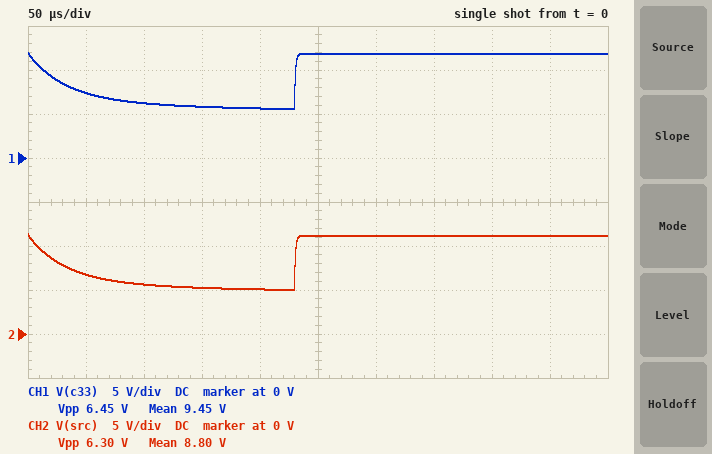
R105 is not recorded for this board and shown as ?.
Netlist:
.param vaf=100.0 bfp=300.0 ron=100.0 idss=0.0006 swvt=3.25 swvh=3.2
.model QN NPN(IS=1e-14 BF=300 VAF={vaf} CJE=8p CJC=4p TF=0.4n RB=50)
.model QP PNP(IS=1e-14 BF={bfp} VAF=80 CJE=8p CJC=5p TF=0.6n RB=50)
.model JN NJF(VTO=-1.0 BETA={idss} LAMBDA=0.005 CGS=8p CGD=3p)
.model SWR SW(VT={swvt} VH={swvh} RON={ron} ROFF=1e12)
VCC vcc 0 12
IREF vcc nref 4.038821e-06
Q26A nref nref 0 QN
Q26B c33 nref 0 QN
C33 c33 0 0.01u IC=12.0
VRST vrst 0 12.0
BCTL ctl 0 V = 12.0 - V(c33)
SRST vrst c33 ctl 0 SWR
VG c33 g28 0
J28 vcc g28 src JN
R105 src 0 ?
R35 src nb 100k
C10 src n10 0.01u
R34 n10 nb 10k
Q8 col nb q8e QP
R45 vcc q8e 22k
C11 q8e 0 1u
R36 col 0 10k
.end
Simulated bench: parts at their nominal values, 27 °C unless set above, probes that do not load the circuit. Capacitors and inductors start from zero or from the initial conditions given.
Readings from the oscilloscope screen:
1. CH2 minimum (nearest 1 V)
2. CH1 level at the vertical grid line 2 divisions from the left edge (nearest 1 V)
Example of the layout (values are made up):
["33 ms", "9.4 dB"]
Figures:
["5 V", "6 V"]
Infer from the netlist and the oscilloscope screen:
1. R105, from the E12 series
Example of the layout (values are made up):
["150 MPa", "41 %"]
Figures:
["3.3 kΩ"]
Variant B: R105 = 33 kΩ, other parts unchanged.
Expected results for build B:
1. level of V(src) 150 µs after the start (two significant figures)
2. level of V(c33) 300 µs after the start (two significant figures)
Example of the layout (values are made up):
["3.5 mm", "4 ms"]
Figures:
["12 V", "12 V"]
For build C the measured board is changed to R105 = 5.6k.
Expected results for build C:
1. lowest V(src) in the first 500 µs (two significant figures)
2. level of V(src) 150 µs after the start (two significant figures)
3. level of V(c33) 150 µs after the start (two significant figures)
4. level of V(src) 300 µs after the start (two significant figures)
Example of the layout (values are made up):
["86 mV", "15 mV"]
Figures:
["8.0 V", "8.8 V", "9.4 V", "8.3 V"]
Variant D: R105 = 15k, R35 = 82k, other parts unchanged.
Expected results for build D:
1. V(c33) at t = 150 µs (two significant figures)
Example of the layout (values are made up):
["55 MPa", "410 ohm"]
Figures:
["12 V"]
